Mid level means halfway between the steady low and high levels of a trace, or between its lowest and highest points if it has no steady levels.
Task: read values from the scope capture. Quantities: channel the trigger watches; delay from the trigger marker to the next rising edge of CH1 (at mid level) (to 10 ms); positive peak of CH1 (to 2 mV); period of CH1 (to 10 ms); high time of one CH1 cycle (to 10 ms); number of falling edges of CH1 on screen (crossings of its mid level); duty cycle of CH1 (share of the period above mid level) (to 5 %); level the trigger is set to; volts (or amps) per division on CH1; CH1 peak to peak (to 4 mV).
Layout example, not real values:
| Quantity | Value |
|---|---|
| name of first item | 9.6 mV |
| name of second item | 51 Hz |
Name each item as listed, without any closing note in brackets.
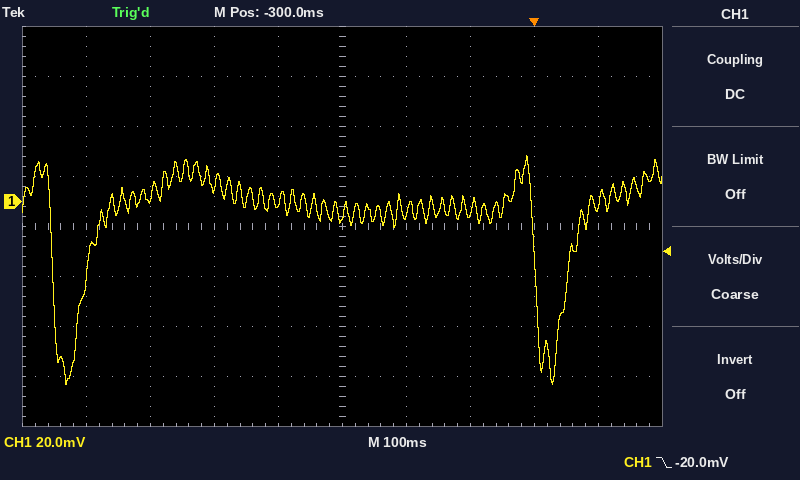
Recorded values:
| Quantity | Value |
|---|---|
| channel the trigger watches | CH1 |
| delay from the trigger marker to the next rising edge of CH1 (at mid level) | 50 ms |
| positive peak of CH1 | 18 mV |
| period of CH1 | 750 ms |
| high time of one CH1 cycle | 700 ms |
| number of falling edges of CH1 on screen | 2 |
| duty cycle of CH1 (share of the period above mid level) | 95 % |
| level the trigger is set to | -20.0 mV |
| volts (or amps) per division on CH1 | 20 mV |
| CH1 peak to peak | 92 mV |
